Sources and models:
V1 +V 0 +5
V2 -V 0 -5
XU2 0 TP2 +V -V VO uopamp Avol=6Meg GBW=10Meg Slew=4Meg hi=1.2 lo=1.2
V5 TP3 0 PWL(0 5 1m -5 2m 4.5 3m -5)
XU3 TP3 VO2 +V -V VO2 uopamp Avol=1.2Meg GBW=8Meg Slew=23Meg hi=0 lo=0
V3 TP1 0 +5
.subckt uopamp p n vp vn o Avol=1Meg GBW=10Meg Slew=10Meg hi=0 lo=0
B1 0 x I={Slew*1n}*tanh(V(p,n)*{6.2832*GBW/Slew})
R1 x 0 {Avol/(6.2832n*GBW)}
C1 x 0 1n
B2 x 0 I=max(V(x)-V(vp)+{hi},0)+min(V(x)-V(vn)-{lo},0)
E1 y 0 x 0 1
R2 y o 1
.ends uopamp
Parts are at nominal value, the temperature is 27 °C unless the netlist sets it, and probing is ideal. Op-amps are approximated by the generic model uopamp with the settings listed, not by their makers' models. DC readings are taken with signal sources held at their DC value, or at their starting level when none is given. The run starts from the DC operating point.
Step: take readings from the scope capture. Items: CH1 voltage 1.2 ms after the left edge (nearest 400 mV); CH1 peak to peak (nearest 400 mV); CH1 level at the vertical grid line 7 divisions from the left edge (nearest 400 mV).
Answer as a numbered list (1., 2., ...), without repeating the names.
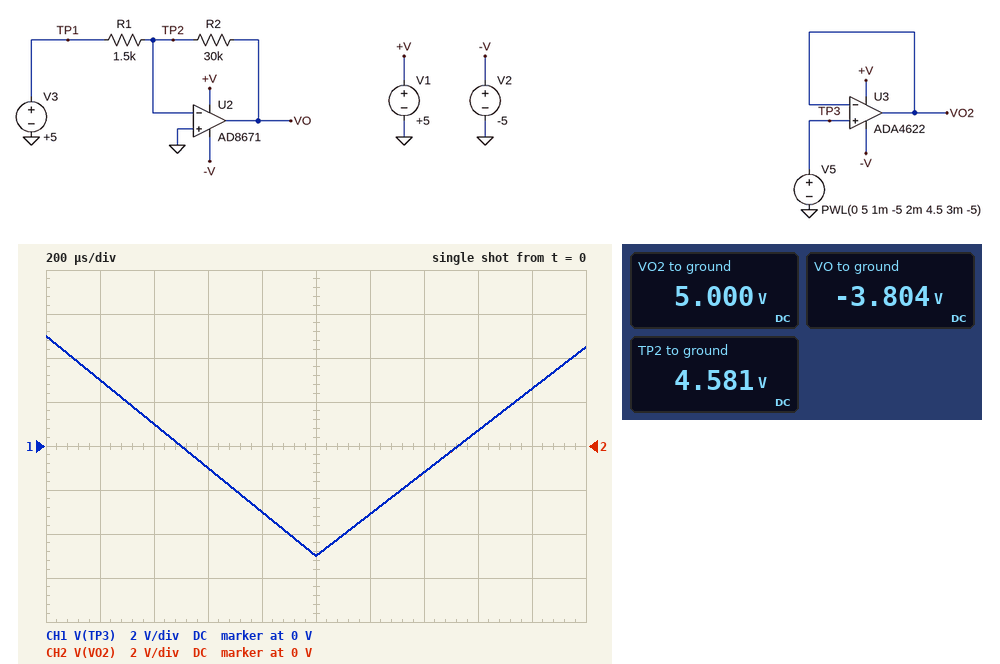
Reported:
1. -3.2 V
2. 10.0 V
3. -1.2 V
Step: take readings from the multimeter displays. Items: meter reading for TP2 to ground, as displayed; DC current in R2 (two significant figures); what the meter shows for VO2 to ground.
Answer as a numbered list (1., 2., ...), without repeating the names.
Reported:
1. 4.581 V
2. 280 µA
3. 5.000 V
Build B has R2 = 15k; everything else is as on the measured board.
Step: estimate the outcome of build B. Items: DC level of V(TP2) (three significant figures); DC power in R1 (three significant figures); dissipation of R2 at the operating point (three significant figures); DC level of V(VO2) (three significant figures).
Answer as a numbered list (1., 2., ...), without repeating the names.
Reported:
1. 4.20 V
2. 427 µW
3. 4.27 mW
4. 5.00 V
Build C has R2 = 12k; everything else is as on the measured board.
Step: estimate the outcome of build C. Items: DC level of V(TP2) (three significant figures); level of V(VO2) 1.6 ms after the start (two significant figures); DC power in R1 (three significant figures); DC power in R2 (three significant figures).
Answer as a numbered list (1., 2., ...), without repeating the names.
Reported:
1. 4.02 V
2. 700 mV
3. 638 µW
4. 5.10 mW
